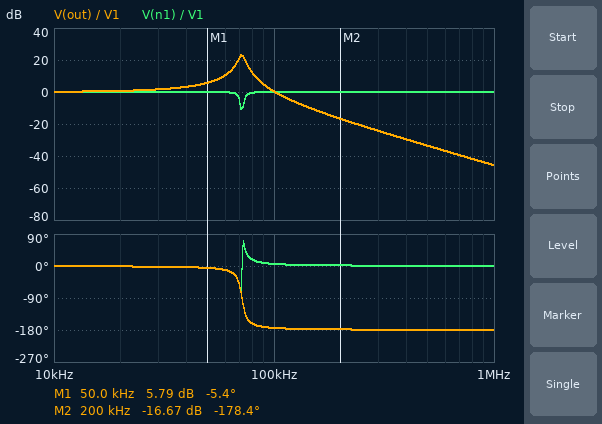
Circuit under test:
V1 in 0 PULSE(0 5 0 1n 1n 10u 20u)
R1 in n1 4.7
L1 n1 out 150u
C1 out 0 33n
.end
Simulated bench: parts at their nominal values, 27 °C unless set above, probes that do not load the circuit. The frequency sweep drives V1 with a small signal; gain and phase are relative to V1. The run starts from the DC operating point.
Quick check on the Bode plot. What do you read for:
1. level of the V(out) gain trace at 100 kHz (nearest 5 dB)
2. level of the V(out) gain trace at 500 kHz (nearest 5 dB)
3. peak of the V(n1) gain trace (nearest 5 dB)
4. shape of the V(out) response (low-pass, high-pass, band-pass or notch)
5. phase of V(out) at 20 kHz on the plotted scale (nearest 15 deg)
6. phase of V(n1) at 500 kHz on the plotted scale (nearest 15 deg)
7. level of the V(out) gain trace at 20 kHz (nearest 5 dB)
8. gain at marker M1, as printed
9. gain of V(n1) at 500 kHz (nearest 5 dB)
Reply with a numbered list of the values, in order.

1. 0 dB
2. -35 dB
3. 0 dB
4. band-pass
5. 0 deg
6. 0 deg
7. 0 dB
8. 5.79 dB
9. 0 dB
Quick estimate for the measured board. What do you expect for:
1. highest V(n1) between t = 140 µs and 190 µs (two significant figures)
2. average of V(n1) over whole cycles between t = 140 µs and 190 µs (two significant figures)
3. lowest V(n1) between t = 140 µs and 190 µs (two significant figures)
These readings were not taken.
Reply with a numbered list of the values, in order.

1. 5.3 V
2. 2.5 V
3. -280 mV
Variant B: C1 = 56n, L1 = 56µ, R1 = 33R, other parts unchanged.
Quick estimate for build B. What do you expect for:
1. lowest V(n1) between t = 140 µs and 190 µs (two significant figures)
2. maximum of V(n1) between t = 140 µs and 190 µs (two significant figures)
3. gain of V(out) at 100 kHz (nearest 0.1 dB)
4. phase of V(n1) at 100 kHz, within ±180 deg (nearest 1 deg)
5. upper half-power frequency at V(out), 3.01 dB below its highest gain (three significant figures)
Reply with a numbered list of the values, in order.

1. -420 mV
2. 5.4 V
3. -1.5 dB
4. 78 deg
5. 104 kHz
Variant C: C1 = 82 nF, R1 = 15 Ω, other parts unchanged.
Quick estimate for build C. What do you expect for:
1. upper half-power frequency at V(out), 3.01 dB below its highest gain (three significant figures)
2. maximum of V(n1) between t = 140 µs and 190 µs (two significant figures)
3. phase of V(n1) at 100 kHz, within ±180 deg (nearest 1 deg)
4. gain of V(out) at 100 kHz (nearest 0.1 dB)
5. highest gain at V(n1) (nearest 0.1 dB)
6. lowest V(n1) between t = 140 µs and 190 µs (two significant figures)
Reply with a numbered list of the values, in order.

1. 51.4 kHz
2. 6.6 V
3. 11 deg
4. -11.9 dB
5. 0 dB
6. -1.6 V
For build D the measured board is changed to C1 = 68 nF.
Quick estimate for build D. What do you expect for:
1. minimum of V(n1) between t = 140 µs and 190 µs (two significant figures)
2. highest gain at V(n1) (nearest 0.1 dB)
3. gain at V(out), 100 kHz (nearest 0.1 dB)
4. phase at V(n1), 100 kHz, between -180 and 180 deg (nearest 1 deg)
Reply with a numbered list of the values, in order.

1. -240 mV
2. 0 dB
3. -9.6 dB
4. 4 deg
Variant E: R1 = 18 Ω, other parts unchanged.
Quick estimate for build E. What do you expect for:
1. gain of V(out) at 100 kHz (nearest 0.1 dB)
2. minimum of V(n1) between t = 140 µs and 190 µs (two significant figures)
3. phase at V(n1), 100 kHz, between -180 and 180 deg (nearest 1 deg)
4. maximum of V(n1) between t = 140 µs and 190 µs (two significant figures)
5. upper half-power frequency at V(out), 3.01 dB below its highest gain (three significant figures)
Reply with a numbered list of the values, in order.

1. -0.2 dB
2. -770 mV
3. 21 deg
4. 5.8 V
5. 79.3 kHz
